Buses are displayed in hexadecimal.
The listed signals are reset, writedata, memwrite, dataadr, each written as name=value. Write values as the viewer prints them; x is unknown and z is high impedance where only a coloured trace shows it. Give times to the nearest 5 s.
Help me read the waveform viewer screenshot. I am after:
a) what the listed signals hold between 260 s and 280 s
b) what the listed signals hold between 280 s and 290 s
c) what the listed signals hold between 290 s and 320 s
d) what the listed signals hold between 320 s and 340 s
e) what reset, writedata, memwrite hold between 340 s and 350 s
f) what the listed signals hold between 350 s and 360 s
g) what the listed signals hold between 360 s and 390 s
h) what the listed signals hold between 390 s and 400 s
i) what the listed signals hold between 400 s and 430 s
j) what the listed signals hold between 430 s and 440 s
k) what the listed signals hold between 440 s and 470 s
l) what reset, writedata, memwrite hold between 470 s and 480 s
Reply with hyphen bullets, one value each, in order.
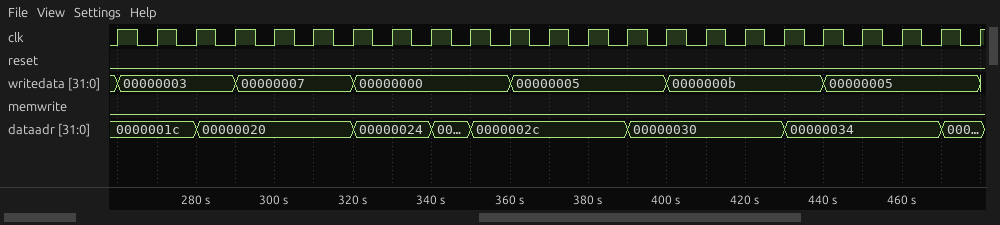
- reset=0, writedata=00000003, memwrite=0, dataadr=0000001c
- reset=0, writedata=00000003, memwrite=0, dataadr=00000020
- reset=0, writedata=00000007, memwrite=0, dataadr=00000020
- reset=0, writedata=00000000, memwrite=0, dataadr=00000024
- reset=0, writedata=00000000, memwrite=0
- reset=0, writedata=00000000, memwrite=0, dataadr=0000002c
- reset=0, writedata=00000005, memwrite=0, dataadr=0000002c
- reset=0, writedata=00000005, memwrite=0, dataadr=00000030
- reset=0, writedata=0000000b, memwrite=0, dataadr=00000030
- reset=0, writedata=0000000b, memwrite=0, dataadr=00000034
- reset=0, writedata=00000005, memwrite=0, dataadr=00000034
- reset=0, writedata=00000005, memwrite=0
